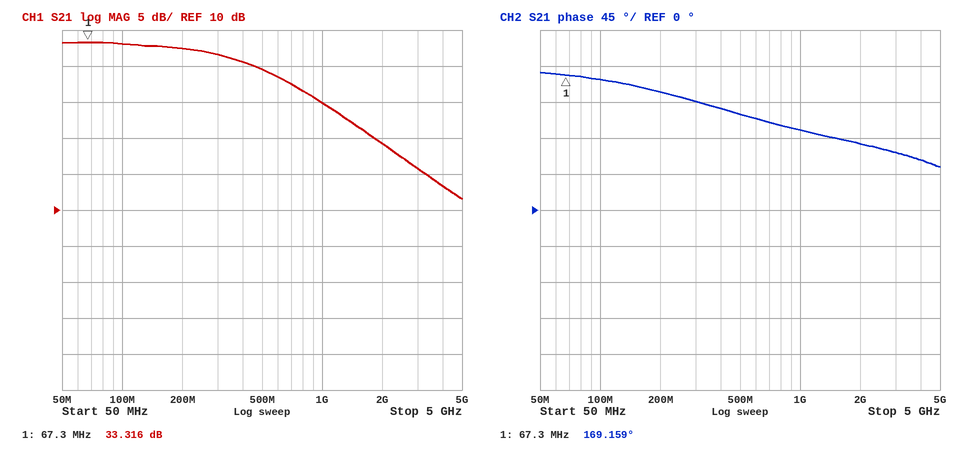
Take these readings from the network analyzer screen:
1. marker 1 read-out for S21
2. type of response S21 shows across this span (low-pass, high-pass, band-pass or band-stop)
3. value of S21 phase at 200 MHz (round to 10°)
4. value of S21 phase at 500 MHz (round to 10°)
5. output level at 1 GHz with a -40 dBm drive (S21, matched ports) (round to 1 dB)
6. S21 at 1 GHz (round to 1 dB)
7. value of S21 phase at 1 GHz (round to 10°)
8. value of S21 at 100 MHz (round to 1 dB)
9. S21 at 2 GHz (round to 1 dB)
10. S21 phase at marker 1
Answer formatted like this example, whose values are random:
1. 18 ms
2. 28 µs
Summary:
1. 33.316 dB
2. low-pass
3. 150°
4. 120°
5. -15 dBm
6. 25 dB
7. 100°
8. 33 dB
9. 19 dB
10. 169.159°
